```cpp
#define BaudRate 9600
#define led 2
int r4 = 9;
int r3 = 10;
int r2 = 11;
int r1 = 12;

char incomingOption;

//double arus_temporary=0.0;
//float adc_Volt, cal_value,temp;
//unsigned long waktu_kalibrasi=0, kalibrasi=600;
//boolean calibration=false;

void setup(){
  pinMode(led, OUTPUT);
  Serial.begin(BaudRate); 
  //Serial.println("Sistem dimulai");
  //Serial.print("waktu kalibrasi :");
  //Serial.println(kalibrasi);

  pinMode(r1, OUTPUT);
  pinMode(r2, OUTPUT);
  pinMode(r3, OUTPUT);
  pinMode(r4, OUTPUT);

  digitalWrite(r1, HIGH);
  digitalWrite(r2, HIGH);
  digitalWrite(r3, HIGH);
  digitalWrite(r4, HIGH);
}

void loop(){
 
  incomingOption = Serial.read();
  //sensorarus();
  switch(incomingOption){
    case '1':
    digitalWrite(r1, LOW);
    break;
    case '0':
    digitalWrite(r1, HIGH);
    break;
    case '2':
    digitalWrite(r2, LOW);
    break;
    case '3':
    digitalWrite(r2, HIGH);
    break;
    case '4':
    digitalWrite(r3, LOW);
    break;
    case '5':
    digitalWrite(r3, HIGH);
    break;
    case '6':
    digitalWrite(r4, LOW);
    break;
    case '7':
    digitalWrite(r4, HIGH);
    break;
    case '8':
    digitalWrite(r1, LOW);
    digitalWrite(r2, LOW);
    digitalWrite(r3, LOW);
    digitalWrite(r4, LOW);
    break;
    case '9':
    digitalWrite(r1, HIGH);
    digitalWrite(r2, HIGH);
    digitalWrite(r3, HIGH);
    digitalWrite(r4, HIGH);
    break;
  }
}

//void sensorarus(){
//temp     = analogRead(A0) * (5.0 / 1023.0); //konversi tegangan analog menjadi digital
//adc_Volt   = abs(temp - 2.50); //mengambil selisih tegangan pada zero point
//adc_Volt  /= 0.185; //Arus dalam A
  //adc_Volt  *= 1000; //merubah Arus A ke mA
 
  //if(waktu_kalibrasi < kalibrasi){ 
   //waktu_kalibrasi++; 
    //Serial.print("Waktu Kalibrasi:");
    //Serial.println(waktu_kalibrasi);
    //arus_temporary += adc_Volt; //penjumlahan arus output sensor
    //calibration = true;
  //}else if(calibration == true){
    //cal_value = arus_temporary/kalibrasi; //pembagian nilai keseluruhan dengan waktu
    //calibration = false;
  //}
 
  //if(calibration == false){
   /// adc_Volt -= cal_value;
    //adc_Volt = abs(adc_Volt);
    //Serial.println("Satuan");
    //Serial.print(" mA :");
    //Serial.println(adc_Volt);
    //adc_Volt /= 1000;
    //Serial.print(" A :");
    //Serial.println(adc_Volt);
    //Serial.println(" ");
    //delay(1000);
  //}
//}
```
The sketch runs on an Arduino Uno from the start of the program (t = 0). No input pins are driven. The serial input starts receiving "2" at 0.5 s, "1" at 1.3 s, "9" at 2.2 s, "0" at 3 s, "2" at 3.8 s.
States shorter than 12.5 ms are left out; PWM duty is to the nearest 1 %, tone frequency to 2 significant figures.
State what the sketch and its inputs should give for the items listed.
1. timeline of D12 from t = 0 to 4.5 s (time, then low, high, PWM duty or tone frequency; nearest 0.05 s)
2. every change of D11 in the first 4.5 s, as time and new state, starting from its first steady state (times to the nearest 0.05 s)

0 s high; 1.3 s low; 2.2 s high
0 s high; 0.5 s low; 2.2 s high; 3.8 s low
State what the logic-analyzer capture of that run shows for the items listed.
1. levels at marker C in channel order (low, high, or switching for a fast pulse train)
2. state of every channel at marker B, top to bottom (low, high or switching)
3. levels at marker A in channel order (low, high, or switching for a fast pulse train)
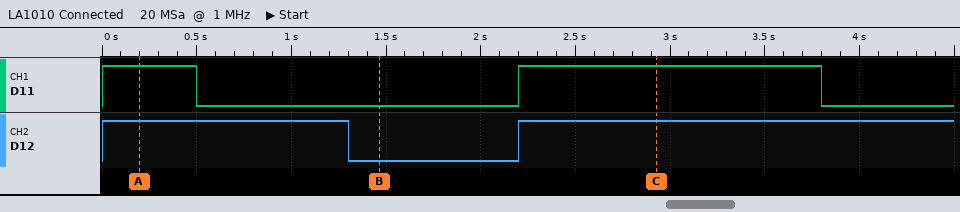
D11 high, D12 high
D11 low, D12 low
D11 high, D12 high
